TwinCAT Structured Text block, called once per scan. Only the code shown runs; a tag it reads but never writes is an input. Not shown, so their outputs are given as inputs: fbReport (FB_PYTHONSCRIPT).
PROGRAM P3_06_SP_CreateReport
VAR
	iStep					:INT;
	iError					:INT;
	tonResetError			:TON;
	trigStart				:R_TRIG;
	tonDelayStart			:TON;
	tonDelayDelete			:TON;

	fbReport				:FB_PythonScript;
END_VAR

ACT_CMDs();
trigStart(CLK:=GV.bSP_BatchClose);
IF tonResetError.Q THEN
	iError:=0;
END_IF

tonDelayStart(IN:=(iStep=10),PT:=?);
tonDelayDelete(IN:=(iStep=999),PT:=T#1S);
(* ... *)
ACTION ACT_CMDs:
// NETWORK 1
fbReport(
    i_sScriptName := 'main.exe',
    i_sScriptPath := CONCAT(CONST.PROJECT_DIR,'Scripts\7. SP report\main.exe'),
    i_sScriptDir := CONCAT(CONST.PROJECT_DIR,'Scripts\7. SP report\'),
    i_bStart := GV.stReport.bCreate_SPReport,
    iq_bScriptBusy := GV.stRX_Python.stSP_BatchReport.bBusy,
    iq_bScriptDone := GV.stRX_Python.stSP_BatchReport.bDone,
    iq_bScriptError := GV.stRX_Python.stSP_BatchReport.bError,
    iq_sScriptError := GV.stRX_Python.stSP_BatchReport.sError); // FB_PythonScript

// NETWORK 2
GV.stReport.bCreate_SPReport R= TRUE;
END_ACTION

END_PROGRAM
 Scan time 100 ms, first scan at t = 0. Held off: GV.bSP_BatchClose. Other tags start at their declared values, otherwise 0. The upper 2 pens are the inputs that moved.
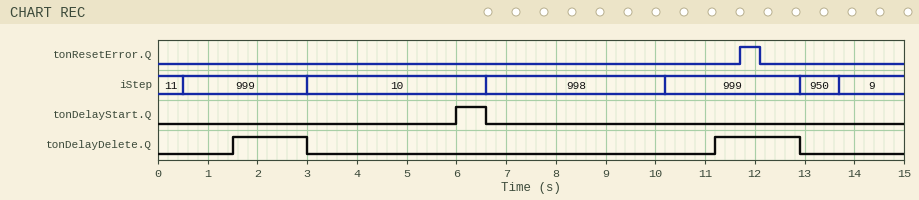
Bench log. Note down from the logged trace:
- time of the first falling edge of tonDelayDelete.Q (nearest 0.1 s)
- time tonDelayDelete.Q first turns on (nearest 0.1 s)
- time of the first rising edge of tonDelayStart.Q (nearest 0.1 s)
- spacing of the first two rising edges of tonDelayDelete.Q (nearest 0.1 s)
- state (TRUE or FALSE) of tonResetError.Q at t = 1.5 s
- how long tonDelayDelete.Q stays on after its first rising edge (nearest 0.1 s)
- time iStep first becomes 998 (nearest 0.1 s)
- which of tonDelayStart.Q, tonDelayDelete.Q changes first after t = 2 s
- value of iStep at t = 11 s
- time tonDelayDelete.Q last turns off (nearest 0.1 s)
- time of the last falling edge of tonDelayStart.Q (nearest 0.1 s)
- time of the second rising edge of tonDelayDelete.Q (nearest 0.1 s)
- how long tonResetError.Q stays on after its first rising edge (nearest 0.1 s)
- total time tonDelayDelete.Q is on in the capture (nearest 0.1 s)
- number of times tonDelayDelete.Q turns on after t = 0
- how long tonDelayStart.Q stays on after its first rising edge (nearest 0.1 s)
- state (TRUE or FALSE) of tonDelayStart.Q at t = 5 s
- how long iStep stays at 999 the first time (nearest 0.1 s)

3.0 s
1.5 s
6.0 s
9.7 s
FALSE
1.5 s
6.6 s
tonDelayDelete.Q
999
12.9 s
6.6 s
11.2 s
0.4 s
3.2 s
2
0.6 s
FALSE
2.5 s
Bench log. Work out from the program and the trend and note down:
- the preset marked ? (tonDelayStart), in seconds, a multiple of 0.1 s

3.0 s
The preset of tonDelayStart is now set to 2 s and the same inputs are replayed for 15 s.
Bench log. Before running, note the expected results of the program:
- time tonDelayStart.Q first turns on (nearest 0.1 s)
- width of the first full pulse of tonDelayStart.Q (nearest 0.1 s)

5.0 s
1.6 s
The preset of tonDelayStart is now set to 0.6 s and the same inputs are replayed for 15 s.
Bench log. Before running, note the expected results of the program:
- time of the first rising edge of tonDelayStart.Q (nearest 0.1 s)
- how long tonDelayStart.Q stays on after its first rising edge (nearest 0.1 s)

3.6 s
3.0 s
